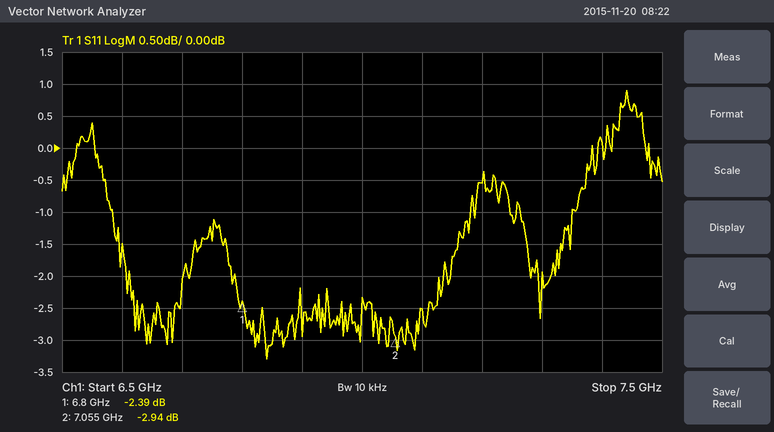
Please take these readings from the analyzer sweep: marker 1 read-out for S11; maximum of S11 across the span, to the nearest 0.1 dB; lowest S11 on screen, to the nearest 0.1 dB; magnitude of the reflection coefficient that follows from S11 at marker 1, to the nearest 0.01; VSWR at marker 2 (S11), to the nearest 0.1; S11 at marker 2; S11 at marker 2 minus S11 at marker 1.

-2.39 dB
0.9 dB
-3.3 dB
0.76
6.0
-2.94 dB
-0.55 dB
